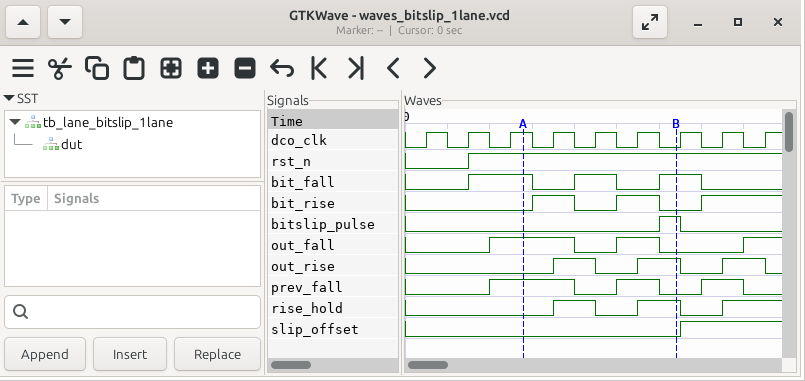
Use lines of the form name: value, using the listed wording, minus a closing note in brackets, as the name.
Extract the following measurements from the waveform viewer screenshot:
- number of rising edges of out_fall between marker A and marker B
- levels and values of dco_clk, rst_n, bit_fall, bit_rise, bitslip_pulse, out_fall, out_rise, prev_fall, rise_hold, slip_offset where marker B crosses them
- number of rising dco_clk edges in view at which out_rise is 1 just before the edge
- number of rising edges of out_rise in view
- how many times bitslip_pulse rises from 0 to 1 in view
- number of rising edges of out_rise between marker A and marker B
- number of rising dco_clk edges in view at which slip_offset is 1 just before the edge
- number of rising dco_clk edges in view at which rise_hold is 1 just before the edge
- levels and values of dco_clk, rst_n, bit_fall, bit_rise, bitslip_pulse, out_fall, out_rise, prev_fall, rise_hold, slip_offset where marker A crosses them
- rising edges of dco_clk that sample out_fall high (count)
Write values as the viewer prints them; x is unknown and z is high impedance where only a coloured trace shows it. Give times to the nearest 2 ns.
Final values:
number of rising edges of out_fall between marker A and marker B: 1
levels and values of dco_clk, rst_n, bit_fall, bit_rise, bitslip_pulse, out_fall, out_rise, prev_fall, rise_hold, slip_offset where marker B crosses them: dco_clk=0, rst_n=1, bit_fall=1, bit_rise=0, bitslip_pulse=1, out_fall=0, out_rise=1, prev_fall=0, rise_hold=1, slip_offset=0
number of rising dco_clk edges in view at which out_rise is 1 just before the edge: 3
number of rising edges of out_rise in view: 3
how many times bitslip_pulse rises from 0 to 1 in view: 1
number of rising edges of out_rise between marker A and marker B: 2
number of rising dco_clk edges in view at which slip_offset is 1 just before the edge: 2
number of rising dco_clk edges in view at which rise_hold is 1 just before the edge: 3
levels and values of dco_clk, rst_n, bit_fall, bit_rise, bitslip_pulse, out_fall, out_rise, prev_fall, rise_hold, slip_offset where marker A crosses them: dco_clk=1, rst_n=1, bit_fall=1, bit_rise=0, bitslip_pulse=0, out_fall=1, out_rise=0, prev_fall=1, rise_hold=0, slip_offset=0
rising edges of dco_clk that sample out_fall high: 4
